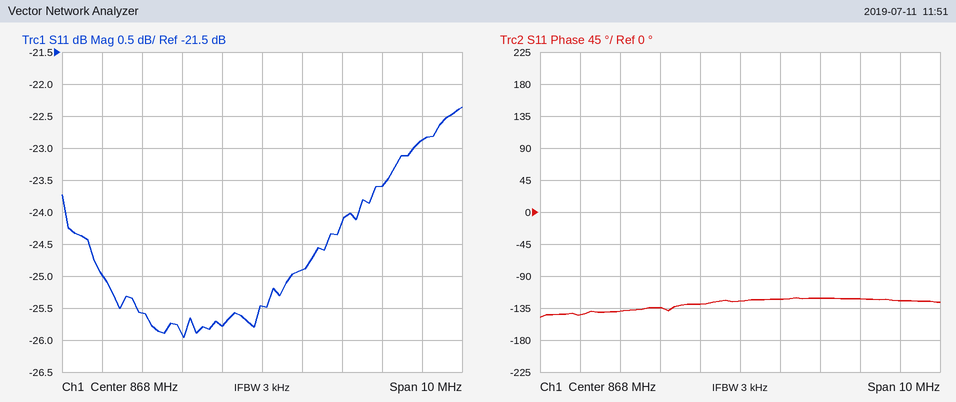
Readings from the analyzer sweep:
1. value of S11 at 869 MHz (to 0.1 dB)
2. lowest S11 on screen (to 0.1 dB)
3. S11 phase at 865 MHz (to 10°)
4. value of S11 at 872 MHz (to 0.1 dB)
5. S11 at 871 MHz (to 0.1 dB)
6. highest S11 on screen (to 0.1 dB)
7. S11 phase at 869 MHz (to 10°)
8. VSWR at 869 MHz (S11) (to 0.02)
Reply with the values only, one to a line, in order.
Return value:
-24.9 dB
-26.0 dB
-140°
-22.9 dB
-23.6 dB
-22.4 dB
-120°
1.12
